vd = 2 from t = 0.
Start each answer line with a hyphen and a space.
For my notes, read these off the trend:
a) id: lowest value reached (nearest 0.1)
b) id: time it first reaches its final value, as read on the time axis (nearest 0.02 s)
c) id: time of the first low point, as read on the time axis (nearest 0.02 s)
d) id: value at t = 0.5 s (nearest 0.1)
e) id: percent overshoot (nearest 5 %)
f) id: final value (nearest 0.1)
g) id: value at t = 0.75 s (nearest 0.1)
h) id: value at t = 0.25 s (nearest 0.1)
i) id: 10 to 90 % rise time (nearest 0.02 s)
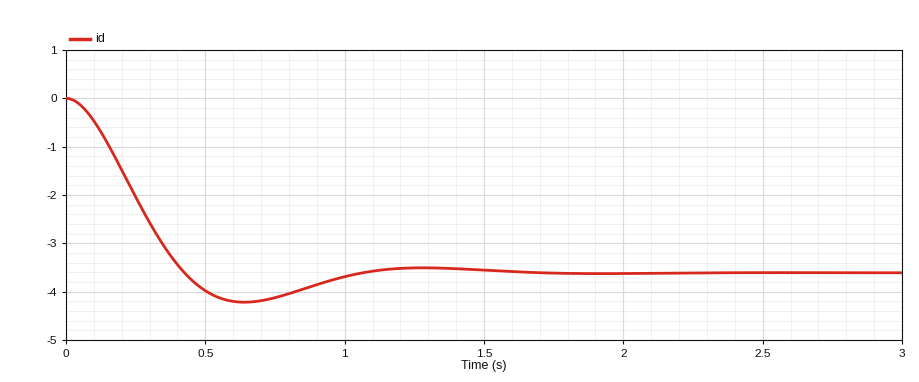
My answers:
- -4.2
- 0.42 s
- 0.64 s
- -4.0
- 15 %
- -3.6
- -4.1
- -2.0
- 0.28 s
